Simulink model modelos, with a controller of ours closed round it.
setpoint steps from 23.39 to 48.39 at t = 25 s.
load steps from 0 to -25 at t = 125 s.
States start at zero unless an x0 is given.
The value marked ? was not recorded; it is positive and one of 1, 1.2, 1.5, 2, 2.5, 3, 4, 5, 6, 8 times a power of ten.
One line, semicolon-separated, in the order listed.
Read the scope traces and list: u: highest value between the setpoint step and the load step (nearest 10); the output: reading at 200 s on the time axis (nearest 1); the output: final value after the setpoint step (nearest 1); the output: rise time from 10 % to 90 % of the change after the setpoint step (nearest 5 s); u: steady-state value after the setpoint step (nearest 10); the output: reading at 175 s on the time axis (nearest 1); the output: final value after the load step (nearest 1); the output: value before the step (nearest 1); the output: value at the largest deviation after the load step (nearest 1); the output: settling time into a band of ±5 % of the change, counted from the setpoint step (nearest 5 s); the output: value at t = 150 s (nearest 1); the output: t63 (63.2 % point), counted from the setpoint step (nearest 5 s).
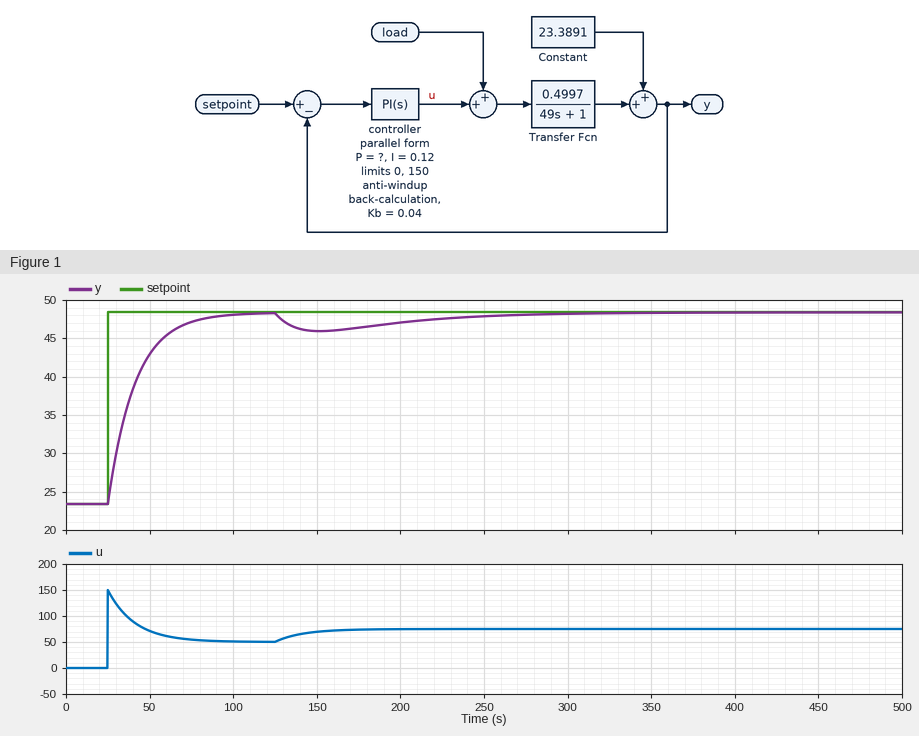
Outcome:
150; 47; 48; 35 s; 50; 46; 48; 23; 46; 50 s; 46; 15 s
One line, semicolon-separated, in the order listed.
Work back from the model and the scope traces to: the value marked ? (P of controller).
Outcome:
6
